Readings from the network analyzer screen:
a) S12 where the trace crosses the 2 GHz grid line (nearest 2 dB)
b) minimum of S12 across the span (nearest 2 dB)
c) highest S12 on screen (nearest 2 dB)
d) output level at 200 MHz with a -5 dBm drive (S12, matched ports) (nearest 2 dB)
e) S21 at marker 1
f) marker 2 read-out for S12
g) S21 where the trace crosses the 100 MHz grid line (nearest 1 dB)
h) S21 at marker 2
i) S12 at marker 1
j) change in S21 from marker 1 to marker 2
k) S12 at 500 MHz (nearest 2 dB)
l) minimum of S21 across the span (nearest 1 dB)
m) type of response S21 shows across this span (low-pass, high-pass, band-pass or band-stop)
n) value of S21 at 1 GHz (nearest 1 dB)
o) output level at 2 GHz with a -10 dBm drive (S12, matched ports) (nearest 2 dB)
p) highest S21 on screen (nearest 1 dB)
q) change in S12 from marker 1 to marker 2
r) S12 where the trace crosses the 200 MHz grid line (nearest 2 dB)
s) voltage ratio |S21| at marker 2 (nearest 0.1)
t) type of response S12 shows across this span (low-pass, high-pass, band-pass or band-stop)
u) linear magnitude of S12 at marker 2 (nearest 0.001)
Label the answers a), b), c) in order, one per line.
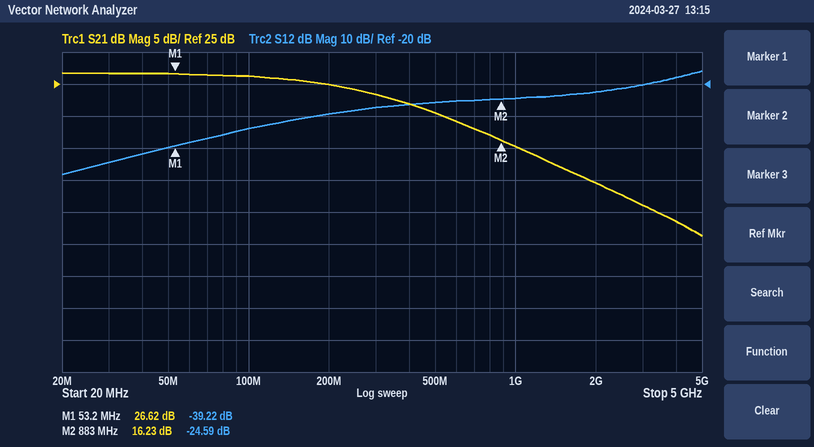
a) -22 dB
b) -48 dB
c) -16 dB
d) -34 dBm
e) 26.62 dB
f) -24.59 dB
g) 26 dB
h) 16.23 dB
i) -39.22 dB
j) -10.39 dB
k) -26 dB
l) 1 dB
m) low-pass
n) 15 dB
o) -32 dBm
p) 27 dB
q) 14.63 dB
r) -30 dB
s) 6.5
t) high-pass
u) 0.059
